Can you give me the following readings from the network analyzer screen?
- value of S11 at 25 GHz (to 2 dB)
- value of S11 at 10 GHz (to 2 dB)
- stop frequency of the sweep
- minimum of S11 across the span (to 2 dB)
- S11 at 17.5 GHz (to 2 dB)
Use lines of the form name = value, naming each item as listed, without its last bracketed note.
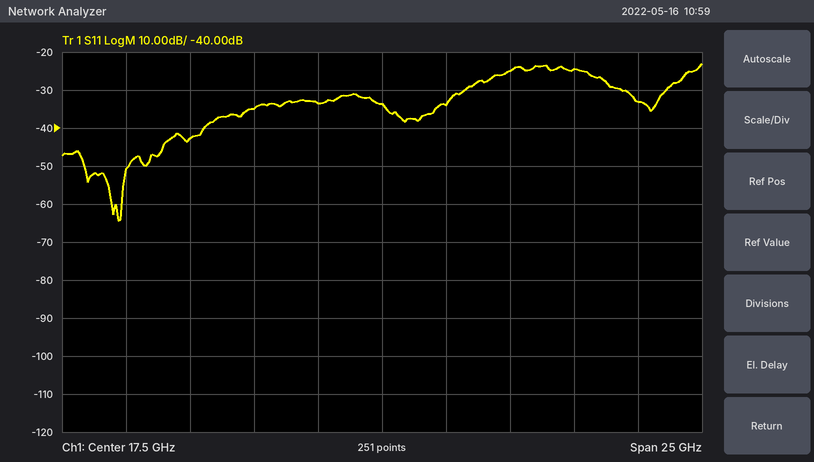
value of S11 at 25 GHz = -24 dB
value of S11 at 10 GHz = -42 dB
stop frequency of the sweep = 30 GHz
minimum of S11 across the span = -64 dB
S11 at 17.5 GHz = -34 dB
